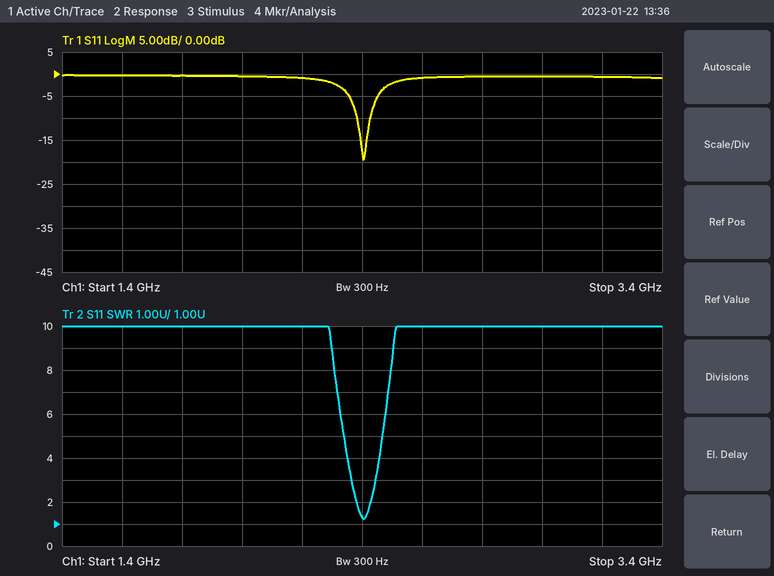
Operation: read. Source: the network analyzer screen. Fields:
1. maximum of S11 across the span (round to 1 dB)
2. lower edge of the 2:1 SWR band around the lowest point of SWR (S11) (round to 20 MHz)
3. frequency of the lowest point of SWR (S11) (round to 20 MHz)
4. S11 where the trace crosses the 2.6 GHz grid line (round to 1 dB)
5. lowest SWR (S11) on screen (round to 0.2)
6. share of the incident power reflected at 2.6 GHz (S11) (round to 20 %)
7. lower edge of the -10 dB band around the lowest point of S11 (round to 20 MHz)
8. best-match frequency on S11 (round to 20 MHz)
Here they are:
0 dB
2.38 GHz
2.40 GHz
-1 dB
1.2
80 %
2.38 GHz
2.40 GHz
